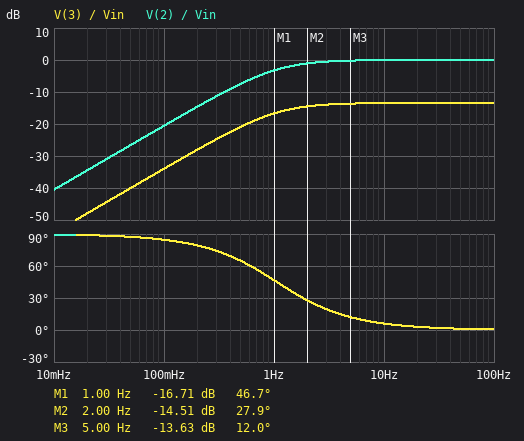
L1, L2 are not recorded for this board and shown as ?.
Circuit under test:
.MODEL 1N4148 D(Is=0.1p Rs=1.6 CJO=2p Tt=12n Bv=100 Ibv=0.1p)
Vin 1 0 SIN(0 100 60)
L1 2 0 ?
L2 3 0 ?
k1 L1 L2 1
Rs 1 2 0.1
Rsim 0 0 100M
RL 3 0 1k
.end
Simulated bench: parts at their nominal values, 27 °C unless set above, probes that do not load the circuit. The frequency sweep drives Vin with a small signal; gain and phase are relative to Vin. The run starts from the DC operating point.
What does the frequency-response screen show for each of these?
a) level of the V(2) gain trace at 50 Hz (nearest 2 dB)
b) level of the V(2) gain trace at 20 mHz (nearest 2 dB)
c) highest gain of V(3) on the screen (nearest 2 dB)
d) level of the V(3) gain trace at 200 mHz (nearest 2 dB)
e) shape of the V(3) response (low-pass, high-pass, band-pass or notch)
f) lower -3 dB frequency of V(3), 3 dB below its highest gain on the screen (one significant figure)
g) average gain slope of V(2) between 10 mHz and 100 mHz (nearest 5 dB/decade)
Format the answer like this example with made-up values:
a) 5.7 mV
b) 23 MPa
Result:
a) 0 dB
b) -34 dB
c) -14 dB
d) -28 dB
e) high-pass
f) 1 Hz
g) 20 dB/decade
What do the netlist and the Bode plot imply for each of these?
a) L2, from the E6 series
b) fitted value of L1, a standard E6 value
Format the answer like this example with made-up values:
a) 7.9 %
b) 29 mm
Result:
a) 680 µH
b) 15 mH
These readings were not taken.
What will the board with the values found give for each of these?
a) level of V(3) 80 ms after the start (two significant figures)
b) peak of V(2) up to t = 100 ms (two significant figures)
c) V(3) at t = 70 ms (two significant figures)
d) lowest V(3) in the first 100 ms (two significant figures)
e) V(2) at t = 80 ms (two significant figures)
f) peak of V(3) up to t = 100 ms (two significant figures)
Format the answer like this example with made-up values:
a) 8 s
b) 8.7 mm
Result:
a) -20 V
b) 99 V
c) 20 V
d) -22 V
e) -96 V
f) 21 V
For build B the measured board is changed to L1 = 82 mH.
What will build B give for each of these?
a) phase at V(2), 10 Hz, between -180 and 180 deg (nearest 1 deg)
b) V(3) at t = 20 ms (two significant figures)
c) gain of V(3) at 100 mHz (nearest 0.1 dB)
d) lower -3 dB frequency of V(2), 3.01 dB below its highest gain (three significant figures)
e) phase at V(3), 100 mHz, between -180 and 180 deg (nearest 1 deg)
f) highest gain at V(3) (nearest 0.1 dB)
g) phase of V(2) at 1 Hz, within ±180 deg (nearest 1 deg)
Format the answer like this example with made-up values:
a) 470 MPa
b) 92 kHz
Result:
a) 1 deg
b) 8.6 V
c) -27.6 dB
d) 194 mHz
e) 63 deg
f) -20.8 dB
g) 11 deg
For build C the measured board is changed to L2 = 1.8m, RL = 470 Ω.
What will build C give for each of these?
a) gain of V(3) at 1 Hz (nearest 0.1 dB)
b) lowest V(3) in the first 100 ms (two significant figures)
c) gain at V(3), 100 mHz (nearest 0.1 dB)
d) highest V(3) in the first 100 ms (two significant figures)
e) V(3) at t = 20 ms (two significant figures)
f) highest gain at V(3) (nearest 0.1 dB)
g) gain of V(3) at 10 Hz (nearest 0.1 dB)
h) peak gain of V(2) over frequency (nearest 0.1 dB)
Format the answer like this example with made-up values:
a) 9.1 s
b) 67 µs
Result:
a) -12.5 dB
b) -35 V
c) -29.8 dB
d) 34 V
e) 33 V
f) -9.2 dB
g) -9.3 dB
h) 0 dB
